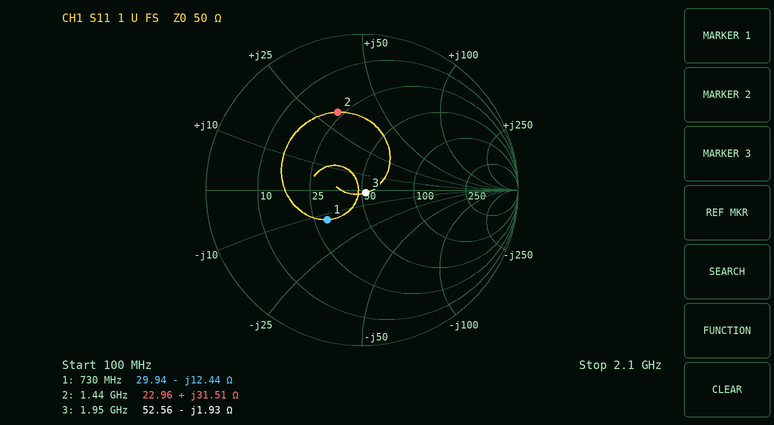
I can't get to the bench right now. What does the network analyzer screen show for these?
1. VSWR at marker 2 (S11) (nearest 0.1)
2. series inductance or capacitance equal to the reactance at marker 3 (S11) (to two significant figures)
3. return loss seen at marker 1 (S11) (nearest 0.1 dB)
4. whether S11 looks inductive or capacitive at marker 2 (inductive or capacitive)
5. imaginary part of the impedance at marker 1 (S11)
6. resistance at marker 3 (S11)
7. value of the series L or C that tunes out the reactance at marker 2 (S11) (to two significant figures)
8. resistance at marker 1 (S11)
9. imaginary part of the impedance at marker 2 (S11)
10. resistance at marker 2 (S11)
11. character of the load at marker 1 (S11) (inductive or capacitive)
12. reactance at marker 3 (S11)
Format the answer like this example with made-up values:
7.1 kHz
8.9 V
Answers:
3.2
42 pF
10.7 dB
inductive
-12.44 Ω
52.56 Ω
3.5 pF
29.94 Ω
+31.51 Ω
22.96 Ω
capacitive
-1.93 Ω
